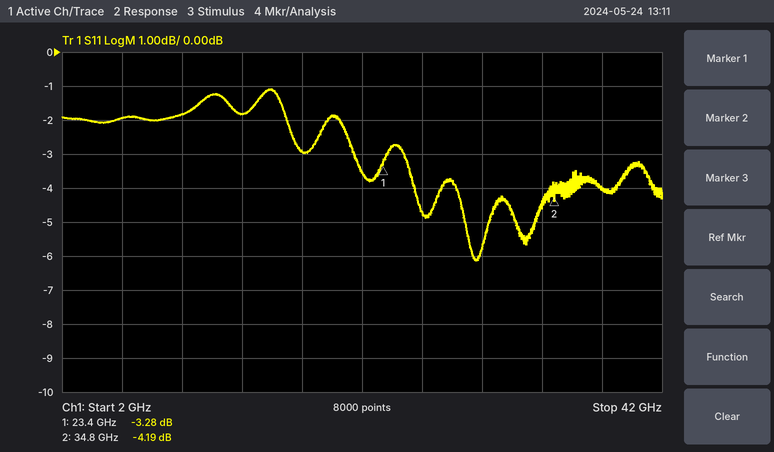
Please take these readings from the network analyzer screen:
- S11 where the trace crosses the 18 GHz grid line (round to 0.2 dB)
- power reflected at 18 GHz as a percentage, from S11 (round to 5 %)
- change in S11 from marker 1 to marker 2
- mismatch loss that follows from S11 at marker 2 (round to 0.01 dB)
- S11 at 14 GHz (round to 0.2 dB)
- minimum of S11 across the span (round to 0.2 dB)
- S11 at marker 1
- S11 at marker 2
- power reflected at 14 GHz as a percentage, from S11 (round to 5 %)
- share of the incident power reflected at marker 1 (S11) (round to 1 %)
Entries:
-3.0 dB
50 %
-0.91 dB
2.08 dB
-1.8 dB
-6.2 dB
-3.28 dB
-4.19 dB
65 %
47 %
